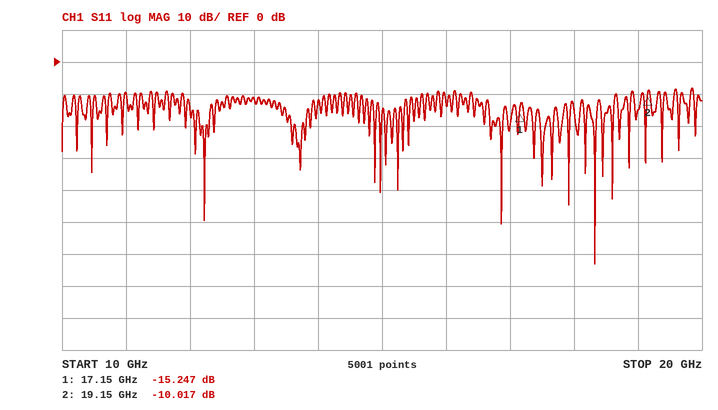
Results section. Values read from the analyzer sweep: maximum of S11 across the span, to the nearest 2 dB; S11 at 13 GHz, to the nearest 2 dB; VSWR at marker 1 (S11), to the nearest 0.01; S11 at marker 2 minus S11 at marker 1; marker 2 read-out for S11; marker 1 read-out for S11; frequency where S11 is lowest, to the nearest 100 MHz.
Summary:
-8 dB
-12 dB
1.42
5.230 dB
-10.017 dB
-15.247 dB
18.3 GHz
